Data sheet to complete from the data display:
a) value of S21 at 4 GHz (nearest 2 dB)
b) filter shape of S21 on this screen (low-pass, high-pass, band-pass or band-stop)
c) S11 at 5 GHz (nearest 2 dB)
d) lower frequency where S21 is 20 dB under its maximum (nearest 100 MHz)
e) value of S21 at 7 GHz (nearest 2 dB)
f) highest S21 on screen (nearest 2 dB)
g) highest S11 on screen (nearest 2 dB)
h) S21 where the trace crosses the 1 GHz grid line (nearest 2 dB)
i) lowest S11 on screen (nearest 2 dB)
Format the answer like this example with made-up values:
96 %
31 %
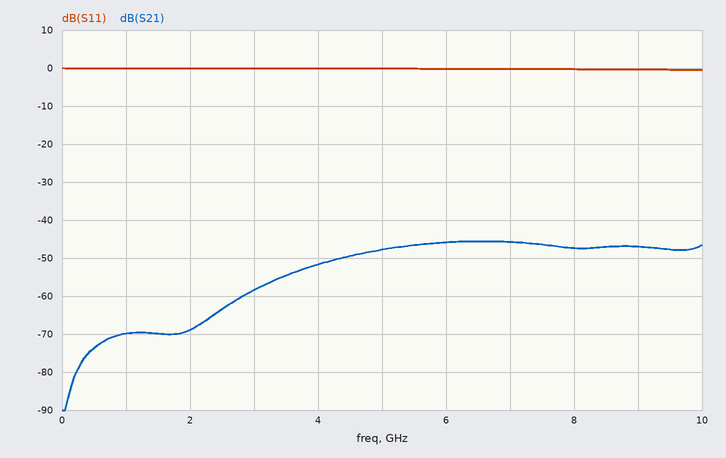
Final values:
-52 dB
high-pass
0 dB
2.3 GHz
-46 dB
-46 dB
0 dB
-70 dB
0 dB
